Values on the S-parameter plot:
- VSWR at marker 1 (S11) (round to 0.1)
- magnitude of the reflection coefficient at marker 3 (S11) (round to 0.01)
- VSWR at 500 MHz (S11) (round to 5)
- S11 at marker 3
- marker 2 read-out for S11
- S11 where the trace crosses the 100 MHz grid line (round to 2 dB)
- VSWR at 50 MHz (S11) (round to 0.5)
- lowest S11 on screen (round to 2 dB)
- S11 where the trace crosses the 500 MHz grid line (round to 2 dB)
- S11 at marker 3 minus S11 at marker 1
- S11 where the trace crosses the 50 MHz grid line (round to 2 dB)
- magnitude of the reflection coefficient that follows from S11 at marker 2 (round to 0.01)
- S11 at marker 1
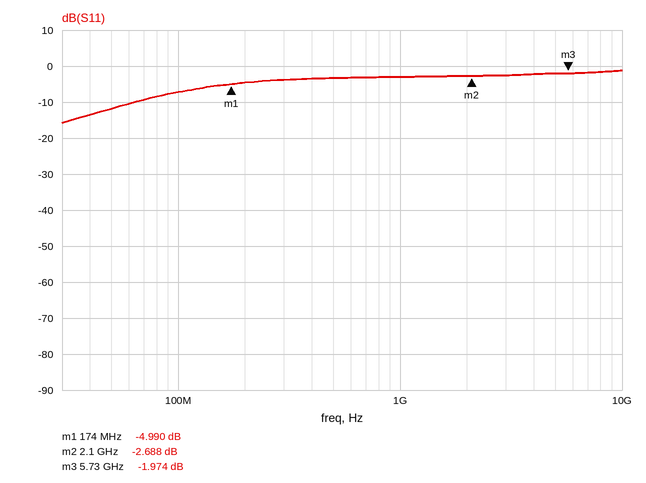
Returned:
3.6
0.80
5
-1.974 dB
-2.688 dB
-8 dB
1.5
-16 dB
-4 dB
3.016 dB
-12 dB
0.73
-4.990 dB
